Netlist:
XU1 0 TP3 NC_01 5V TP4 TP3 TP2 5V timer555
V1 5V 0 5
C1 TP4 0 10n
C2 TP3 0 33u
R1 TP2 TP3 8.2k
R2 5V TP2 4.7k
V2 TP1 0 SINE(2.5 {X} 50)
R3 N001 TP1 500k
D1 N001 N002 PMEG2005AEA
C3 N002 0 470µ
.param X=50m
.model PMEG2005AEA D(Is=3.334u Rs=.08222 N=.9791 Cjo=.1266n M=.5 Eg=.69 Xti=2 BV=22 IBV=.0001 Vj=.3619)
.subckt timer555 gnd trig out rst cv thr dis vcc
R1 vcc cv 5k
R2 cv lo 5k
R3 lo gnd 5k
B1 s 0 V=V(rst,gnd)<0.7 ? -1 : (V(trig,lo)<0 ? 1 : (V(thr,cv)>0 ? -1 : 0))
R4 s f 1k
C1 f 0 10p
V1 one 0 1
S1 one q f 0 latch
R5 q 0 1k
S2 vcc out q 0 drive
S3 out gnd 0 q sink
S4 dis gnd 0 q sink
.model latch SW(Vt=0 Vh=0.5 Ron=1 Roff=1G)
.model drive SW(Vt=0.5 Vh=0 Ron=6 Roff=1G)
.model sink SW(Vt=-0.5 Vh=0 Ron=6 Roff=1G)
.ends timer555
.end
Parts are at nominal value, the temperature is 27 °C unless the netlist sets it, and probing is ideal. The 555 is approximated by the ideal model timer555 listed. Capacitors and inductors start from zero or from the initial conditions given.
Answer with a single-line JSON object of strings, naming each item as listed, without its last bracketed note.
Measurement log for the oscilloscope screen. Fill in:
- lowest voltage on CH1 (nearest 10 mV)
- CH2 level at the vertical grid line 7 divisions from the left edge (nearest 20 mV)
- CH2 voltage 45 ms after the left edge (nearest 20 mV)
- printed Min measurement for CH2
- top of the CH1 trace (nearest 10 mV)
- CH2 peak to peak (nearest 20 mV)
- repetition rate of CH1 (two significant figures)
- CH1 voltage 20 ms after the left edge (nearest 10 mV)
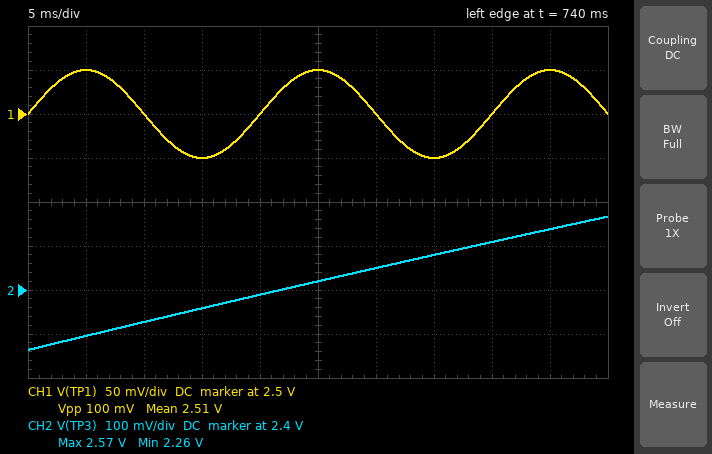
{"lowest voltage on CH1": "2.45 V", "CH2 level at the vertical grid line 7 divisions from the left edge": "2.48 V", "CH2 voltage 45 ms after the left edge": "2.54 V", "printed Min measurement for CH2": "2.26 V", "top of the CH1 trace": "2.55 V", "CH2 peak to peak": "300 mV", "repetition rate of CH1": "50 Hz", "CH1 voltage 20 ms after the left edge": "2.50 V"}
